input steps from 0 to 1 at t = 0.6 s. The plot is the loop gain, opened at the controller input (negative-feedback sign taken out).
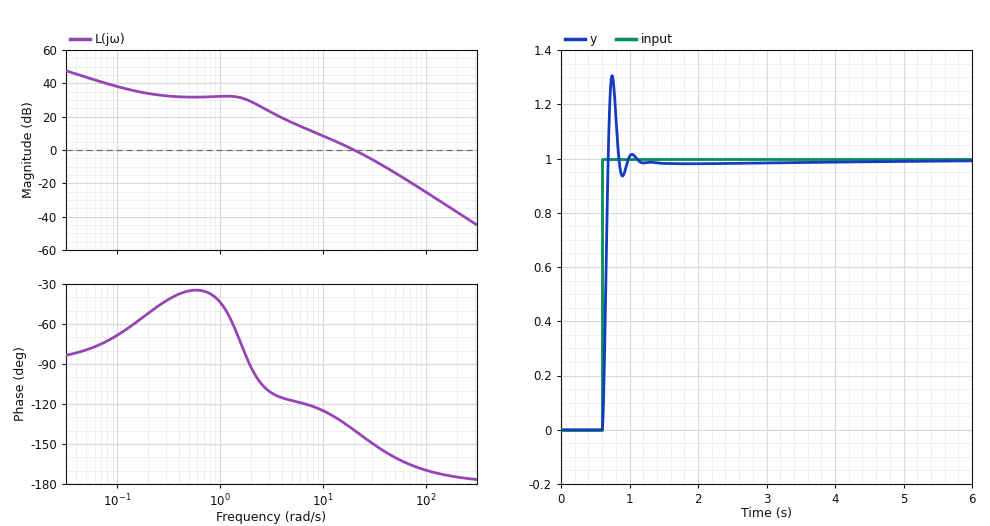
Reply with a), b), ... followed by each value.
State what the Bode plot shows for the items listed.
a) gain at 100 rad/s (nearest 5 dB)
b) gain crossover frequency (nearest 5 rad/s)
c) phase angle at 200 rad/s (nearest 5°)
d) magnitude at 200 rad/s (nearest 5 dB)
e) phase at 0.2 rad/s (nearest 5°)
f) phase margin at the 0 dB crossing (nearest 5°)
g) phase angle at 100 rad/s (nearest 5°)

a) -25 dB
b) 20 rad/s
c) -175°
d) -35 dB
e) -50°
f) 40°
g) -170°
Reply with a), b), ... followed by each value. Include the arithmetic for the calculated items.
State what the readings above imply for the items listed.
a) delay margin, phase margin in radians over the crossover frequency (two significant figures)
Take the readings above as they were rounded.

a) 40 × π / 180 / 20 = 0.035 s
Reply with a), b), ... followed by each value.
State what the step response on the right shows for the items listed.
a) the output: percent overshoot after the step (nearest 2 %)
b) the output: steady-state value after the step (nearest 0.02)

a) 30 %
b) 1.00
